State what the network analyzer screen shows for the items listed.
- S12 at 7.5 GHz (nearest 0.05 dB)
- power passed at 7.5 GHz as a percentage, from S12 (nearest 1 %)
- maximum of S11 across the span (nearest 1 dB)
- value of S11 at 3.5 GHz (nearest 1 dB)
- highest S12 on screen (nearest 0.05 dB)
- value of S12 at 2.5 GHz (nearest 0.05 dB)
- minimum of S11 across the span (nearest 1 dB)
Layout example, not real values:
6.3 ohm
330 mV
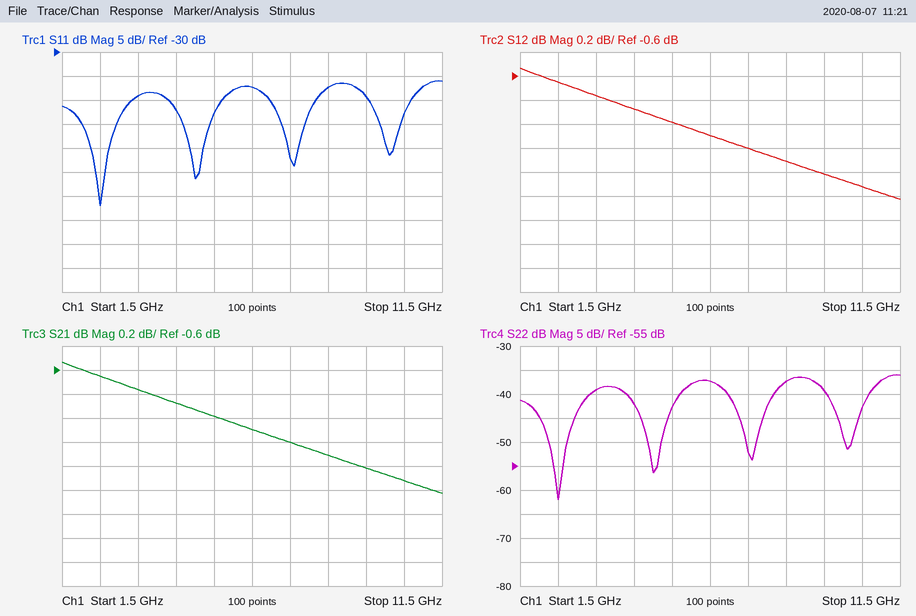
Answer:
-1.20 dB
76 %
-36 dB
-39 dB
-0.55 dB
-0.65 dB
-62 dB
